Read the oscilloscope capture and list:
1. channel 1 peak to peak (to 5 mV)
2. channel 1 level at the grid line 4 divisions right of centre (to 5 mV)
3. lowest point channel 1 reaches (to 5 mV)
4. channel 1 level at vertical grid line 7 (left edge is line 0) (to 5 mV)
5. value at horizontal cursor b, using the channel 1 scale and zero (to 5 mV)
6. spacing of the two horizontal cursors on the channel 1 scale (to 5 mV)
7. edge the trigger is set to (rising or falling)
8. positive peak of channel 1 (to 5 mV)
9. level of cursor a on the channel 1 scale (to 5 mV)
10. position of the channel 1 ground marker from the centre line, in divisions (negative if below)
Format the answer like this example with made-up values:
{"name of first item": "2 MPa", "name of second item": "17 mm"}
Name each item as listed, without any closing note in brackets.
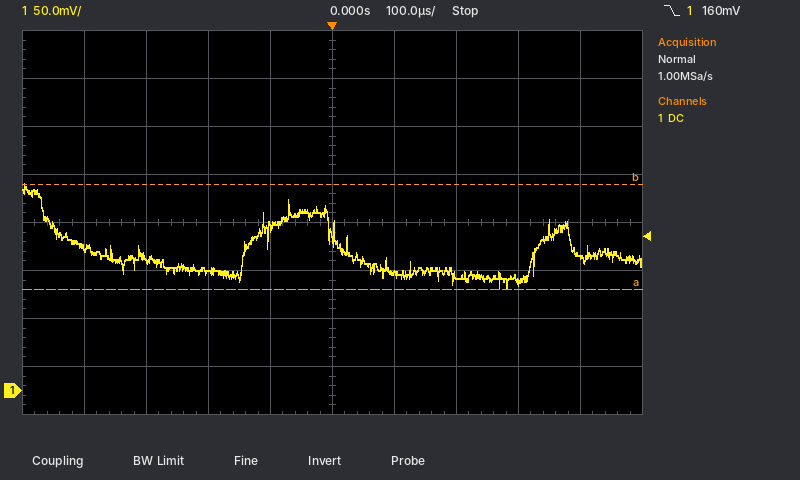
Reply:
{"channel 1 peak to peak": "110 mV", "channel 1 level at the grid line 4 divisions right of centre": "140 mV", "lowest point channel 1 reaches": "105 mV", "channel 1 level at vertical grid line 7 (left edge is line 0)": "120 mV", "value at horizontal cursor b, using the channel 1 scale and zero": "215 mV", "spacing of the two horizontal cursors on the channel 1 scale": "110 mV", "edge the trigger is set to": "falling", "positive peak of channel 1": "215 mV", "level of cursor a on the channel 1 scale": "105 mV", "position of the channel 1 ground marker from the centre line, in divisions": "-3.5 div"}
